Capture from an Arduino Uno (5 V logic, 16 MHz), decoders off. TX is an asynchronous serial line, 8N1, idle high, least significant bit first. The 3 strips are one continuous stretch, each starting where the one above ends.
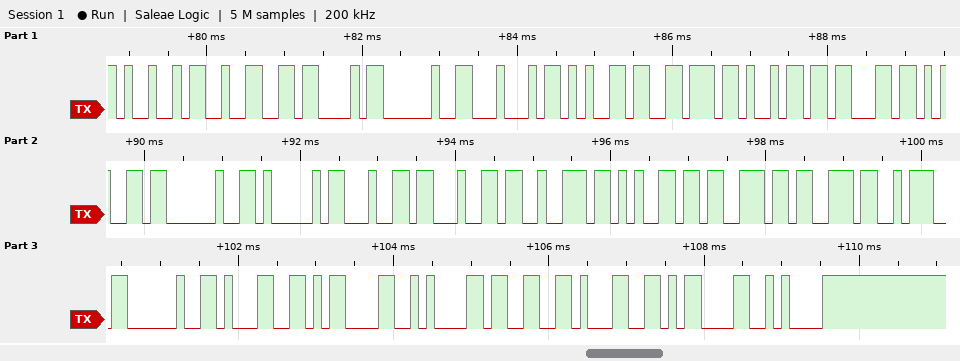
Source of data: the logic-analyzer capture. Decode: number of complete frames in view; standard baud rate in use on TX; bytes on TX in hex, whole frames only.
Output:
27
9600 baud
0x49 0x32 0x43 0x20 0x44 0x65 0x76 0x69 0x63 0x65 0x20 0x41 0x64 0x64 0x72 0x65 0x73 0x73 0x3A 0x20 0x31 0x0D 0x0A 0x33 0x31 0x0D 0x0A
